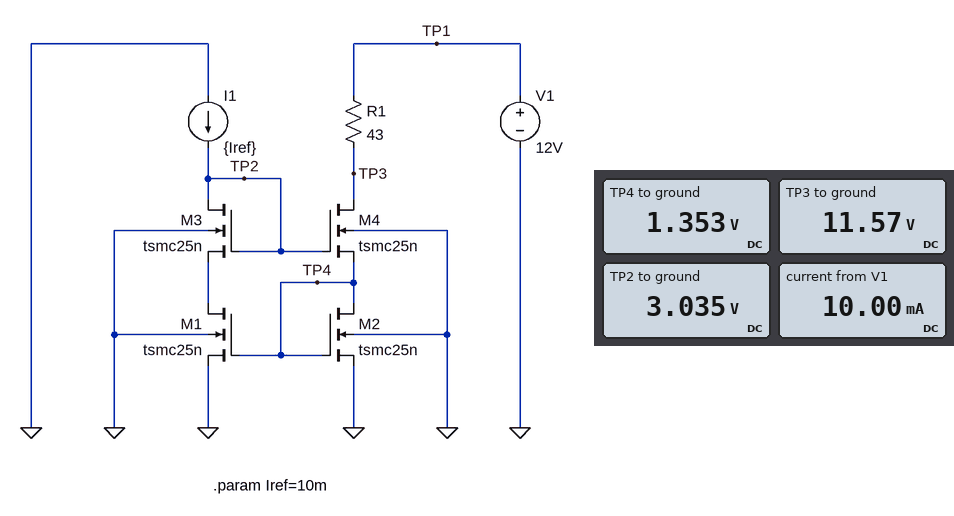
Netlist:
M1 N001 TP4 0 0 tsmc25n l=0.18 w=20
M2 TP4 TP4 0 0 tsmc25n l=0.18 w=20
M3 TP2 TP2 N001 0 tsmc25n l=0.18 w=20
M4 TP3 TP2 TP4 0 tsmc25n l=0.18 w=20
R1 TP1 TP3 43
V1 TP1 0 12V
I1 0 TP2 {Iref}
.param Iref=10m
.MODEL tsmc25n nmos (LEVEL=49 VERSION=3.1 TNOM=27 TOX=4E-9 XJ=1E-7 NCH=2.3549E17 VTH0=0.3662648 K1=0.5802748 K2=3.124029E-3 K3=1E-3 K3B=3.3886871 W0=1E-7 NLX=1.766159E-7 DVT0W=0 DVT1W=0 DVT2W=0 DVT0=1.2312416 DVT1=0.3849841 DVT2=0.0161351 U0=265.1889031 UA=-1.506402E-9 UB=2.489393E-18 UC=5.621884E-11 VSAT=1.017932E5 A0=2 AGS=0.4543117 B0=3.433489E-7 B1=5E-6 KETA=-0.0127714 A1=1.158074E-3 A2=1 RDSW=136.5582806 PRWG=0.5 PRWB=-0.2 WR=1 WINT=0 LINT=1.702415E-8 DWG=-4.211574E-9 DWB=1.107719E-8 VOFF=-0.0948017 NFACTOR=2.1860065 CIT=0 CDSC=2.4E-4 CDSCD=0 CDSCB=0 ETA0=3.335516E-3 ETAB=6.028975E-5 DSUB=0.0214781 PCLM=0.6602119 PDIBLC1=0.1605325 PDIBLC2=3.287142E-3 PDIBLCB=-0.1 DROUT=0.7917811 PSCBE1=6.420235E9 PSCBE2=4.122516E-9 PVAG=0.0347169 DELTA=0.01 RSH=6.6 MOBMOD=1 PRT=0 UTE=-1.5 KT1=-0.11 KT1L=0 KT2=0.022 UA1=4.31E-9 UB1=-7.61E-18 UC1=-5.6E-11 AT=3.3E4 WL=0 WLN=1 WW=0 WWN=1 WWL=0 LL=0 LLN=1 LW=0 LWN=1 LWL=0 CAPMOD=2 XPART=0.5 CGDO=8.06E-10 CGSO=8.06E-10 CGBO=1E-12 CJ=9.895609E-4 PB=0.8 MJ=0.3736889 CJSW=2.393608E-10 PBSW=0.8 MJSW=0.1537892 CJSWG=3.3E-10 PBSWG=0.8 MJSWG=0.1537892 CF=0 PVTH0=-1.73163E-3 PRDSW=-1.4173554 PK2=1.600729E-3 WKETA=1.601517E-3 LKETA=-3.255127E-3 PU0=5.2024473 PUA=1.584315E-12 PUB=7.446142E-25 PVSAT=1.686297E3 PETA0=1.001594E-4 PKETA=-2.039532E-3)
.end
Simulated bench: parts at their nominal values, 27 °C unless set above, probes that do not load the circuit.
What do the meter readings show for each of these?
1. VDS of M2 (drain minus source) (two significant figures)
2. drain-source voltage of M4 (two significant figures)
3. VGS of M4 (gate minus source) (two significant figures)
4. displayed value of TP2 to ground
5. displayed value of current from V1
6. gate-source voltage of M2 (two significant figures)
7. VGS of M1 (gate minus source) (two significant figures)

1.4 V
10 V
1.7 V
3.035 V
10.00 mA
1.4 V
1.4 V
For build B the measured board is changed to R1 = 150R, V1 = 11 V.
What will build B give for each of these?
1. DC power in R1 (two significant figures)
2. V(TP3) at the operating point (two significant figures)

15 mW
9.5 V
